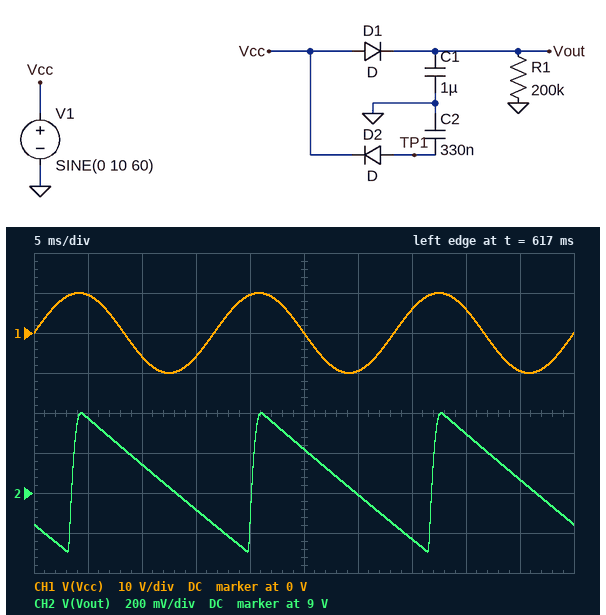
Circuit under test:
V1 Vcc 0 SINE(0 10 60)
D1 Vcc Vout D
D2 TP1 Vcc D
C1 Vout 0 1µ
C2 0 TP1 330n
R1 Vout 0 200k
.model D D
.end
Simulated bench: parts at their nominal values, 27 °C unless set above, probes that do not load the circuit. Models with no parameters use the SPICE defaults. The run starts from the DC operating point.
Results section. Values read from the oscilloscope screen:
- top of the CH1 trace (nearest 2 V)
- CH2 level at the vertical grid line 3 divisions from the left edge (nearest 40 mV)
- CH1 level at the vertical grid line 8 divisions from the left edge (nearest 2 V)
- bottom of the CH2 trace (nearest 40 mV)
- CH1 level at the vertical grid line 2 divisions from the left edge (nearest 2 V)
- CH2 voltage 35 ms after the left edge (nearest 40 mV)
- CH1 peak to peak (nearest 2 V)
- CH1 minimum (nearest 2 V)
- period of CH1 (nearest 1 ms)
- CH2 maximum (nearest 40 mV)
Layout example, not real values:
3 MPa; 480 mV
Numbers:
10 V; 8.92 V; 6 V; 8.72 V; -6 V; 8.76 V; 20 V; -10 V; 17 ms; 9.40 V
